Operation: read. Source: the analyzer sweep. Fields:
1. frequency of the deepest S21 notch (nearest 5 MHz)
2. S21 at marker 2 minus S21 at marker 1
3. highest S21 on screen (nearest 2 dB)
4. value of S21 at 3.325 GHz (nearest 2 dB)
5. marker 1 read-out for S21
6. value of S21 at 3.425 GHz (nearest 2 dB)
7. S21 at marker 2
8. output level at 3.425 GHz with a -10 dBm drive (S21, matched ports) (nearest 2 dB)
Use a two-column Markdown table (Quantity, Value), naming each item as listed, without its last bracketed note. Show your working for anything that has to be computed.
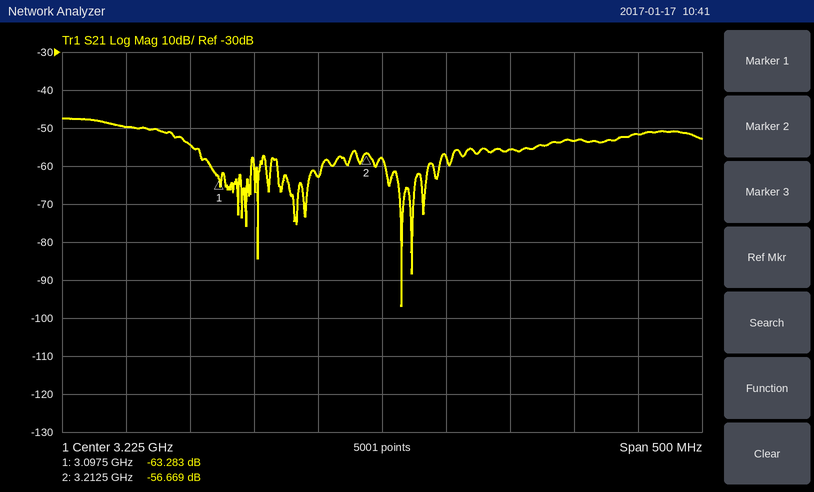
| Quantity | Value |
|---|---|
| frequency of the deepest S21 notch | 3.240 GHz |
| S21 at marker 2 minus S21 at marker 1 | -56.669 − (-63.283) = 6.614 dB |
| highest S21 on screen | -48 dB |
| value of S21 at 3.325 GHz | -56 dB |
| marker 1 read-out for S21 | -63.283 dB |
| value of S21 at 3.425 GHz | -52 dB |
| S21 at marker 2 | -56.669 dB |
| output level at 3.425 GHz with a -10 dBm drive (S21, matched ports) | -10 dBm + (-52 dB) = -62 dBm |
